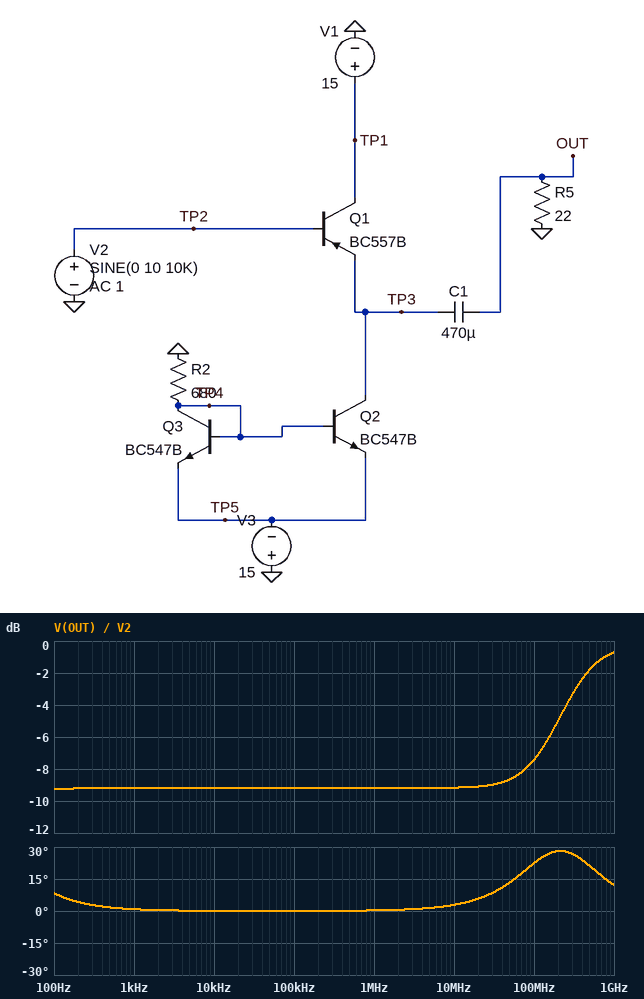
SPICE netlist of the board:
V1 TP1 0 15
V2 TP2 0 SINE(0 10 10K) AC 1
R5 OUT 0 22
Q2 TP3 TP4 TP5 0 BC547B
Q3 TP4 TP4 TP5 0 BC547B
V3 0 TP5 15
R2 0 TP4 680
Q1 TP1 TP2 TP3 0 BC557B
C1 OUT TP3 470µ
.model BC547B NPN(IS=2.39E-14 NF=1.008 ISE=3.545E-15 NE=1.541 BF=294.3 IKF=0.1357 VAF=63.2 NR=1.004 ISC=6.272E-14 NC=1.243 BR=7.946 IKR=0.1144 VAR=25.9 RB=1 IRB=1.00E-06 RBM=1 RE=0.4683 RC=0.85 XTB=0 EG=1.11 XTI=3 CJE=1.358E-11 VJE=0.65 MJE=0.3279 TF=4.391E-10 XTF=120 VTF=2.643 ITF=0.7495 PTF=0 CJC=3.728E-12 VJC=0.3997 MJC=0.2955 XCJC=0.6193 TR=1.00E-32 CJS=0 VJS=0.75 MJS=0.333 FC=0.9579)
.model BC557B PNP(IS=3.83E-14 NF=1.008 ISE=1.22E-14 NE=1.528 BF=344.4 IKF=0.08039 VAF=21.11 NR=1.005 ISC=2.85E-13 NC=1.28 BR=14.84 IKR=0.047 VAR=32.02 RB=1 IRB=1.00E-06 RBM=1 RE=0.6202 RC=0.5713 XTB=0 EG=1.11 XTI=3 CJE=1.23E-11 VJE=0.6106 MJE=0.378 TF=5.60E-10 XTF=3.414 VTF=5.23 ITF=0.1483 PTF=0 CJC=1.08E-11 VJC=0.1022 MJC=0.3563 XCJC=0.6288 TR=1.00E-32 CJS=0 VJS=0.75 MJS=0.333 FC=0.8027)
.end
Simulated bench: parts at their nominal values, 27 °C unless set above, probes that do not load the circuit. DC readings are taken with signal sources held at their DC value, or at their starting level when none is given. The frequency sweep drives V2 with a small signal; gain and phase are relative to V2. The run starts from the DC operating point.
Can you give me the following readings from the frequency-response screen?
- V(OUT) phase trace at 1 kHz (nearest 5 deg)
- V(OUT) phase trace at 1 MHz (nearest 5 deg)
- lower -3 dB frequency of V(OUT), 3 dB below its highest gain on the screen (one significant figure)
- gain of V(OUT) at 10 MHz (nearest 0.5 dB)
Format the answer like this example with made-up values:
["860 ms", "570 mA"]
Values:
["0 deg", "0 deg", "300 MHz", "-9.0 dB"]
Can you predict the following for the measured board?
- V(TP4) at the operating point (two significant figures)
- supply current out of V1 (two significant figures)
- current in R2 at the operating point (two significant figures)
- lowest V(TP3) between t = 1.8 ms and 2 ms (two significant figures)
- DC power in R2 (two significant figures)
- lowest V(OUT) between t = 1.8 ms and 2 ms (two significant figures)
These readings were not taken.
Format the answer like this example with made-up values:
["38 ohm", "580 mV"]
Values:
["-14 V", "9.0 A", "21 mA", "6.4 V", "300 mW", "-3.5 V"]
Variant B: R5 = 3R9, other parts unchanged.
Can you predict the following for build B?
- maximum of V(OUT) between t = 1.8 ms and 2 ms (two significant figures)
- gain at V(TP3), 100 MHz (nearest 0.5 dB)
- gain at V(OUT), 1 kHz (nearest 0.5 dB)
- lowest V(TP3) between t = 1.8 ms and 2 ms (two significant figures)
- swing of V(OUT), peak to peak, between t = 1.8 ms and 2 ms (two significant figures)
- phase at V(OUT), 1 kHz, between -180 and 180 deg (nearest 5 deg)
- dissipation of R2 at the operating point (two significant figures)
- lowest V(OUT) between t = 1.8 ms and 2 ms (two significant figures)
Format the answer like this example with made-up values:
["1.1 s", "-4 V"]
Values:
["2.9 V", "-9.0 dB", "-11.0 dB", "7.0 V", "5.8 V", "5 deg", "300 mW", "-2.9 V"]
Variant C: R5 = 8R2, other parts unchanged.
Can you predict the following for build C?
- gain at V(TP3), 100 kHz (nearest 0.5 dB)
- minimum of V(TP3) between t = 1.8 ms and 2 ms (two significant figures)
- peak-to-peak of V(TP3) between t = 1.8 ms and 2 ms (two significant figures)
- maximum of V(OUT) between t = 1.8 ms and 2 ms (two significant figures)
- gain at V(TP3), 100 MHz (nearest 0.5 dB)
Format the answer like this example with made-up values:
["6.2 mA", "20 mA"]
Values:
["-10.0 dB", "6.6 V", "6.5 V", "3.2 V", "-8.0 dB"]
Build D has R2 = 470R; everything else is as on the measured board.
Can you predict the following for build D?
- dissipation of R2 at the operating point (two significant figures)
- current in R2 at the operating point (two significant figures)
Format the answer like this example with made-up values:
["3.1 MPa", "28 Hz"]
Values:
["430 mW", "30 mA"]
